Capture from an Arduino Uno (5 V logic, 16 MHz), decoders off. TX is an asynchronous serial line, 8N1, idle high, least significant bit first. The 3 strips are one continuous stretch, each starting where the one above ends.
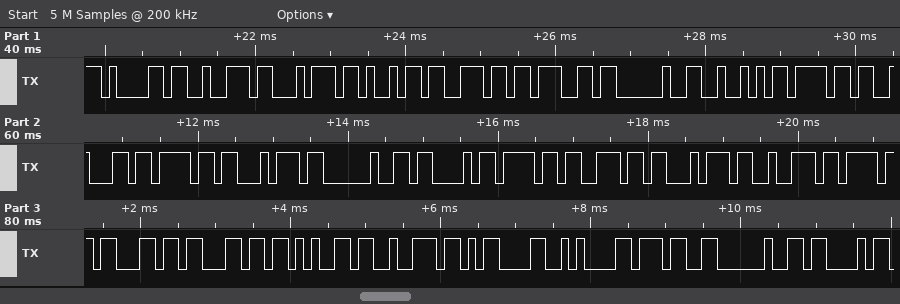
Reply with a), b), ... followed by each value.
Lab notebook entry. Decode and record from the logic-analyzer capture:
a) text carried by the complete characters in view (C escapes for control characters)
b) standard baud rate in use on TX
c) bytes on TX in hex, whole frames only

a) "arting Robot Controller\r\n7 C"
b) 9600 baud
c) 61 72 74 69 6E 67 20 52 6F 62 6F 74 20 43 6F 6E 74 72 6F 6C 6C 65 72 0D 0A 37 20 43
